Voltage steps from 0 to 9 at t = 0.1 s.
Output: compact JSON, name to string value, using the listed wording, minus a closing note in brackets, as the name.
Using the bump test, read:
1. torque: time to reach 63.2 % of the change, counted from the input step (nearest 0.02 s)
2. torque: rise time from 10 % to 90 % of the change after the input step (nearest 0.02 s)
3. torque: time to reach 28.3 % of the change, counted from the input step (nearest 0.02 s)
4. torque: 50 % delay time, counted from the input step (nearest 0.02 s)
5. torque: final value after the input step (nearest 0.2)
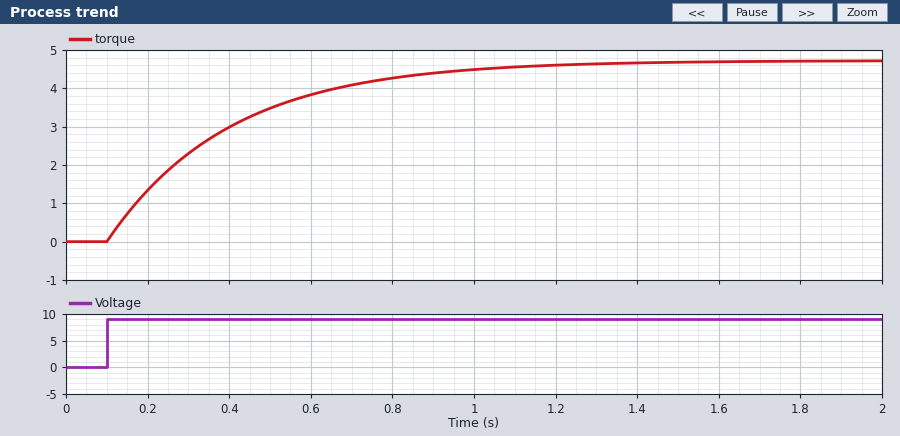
{"torque: time to reach 63.2 % of the change, counted from the input step": "0.30 s", "torque: rise time from 10 % to 90 % of the change after the input step": "0.66 s", "torque: time to reach 28.3 % of the change, counted from the input step": "0.10 s", "torque: 50 % delay time, counted from the input step": "0.20 s", "torque: final value after the input step": "4.8"}
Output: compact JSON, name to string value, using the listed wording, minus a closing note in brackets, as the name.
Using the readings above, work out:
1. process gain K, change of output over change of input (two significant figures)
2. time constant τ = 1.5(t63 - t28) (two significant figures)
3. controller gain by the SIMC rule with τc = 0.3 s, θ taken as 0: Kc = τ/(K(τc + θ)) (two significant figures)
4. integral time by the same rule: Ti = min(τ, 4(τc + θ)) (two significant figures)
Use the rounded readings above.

{"process gain K, change of output over change of input": "0.53", "time constant τ = 1.5(t63 - t28)": "0.30 s", "controller gain by the SIMC rule with τc = 0.3 s, θ taken as 0: Kc = τ/(K(τc + θ))": "1.9", "integral time by the same rule: Ti = min(τ, 4(τc + θ))": "0.30 s"}
